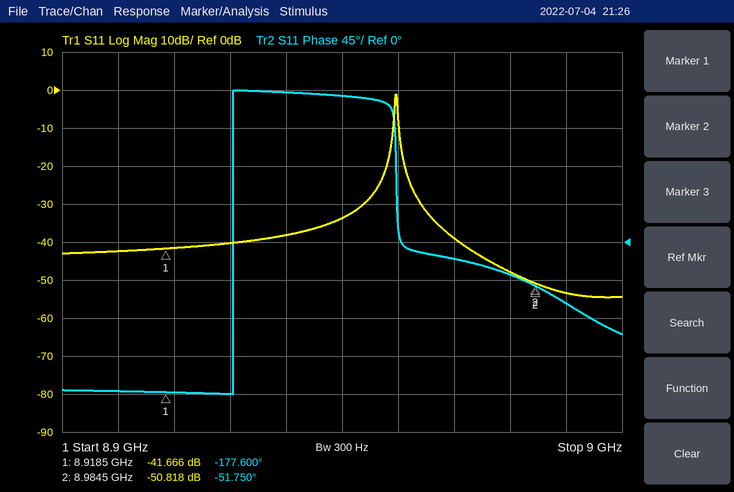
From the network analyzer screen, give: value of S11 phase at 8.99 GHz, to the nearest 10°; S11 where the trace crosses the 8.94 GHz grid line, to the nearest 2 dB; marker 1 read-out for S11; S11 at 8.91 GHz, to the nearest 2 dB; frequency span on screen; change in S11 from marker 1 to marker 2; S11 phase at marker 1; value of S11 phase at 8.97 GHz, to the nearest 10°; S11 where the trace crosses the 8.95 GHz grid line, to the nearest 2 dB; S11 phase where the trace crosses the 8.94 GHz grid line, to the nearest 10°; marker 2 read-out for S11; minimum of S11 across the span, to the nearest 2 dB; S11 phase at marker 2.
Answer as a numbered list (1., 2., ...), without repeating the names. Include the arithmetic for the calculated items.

1. -70°
2. -38 dB
3. -41.666 dB
4. -42 dB
5. 100 MHz
6. -50.818 − (-41.666) = -9.152 dB
7. -177.600°
8. -20°
9. -34 dB
10. 180°
11. -50.818 dB
12. -54 dB
13. -51.750°
